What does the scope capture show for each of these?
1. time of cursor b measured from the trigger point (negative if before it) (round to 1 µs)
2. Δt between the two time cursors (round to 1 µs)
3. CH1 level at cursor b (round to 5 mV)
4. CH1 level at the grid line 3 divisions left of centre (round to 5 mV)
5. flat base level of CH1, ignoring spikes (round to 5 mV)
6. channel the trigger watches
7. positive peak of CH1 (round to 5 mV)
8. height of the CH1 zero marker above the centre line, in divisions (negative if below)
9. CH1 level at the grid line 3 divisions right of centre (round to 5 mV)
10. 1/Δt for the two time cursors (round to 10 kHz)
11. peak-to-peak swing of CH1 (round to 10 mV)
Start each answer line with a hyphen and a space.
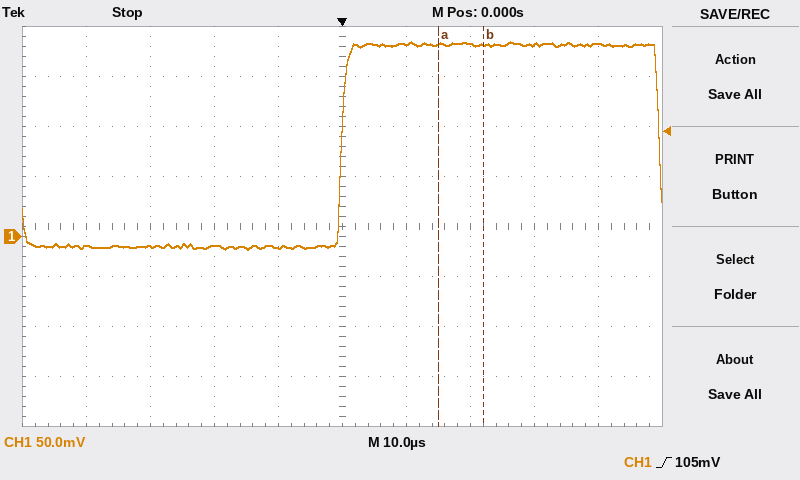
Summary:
- +22 µs
- 7 µs
- 190 mV
- -10 mV
- -10 mV
- CH1
- 195 mV
- -0.2 div
- 190 mV
- 140 kHz
- 210 mV
